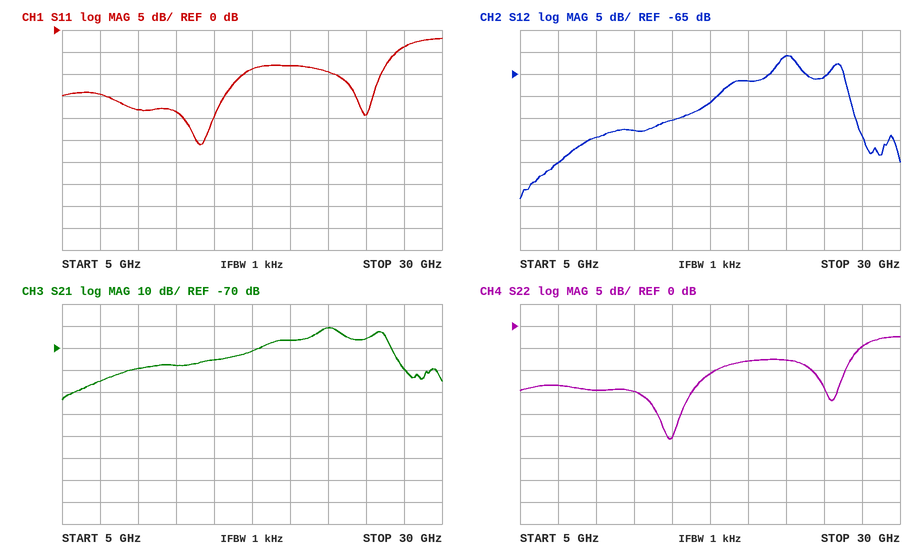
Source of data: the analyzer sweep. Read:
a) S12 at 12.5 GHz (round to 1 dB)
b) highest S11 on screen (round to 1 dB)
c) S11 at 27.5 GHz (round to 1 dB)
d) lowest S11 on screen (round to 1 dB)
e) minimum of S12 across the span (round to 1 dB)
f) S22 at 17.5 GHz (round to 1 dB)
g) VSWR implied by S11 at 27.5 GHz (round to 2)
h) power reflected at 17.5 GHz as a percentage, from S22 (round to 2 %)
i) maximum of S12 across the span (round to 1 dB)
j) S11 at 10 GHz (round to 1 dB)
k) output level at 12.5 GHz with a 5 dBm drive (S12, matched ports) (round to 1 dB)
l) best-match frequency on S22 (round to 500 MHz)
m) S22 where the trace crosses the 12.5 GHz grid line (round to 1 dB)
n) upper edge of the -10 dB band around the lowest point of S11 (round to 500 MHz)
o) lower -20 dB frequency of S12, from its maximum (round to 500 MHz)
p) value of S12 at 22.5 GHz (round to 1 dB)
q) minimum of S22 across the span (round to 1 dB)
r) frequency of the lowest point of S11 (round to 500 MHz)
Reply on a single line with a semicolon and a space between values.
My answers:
-78 dB; -2 dB; -4 dB; -26 dB; -93 dB; -11 dB; 4; 8 %; -61 dB; -18 dB; -73 dBm; 15.0 GHz; -15 dB; 17.0 GHz; 9.0 GHz; -61 dB; -26 dB; 14.0 GHz
